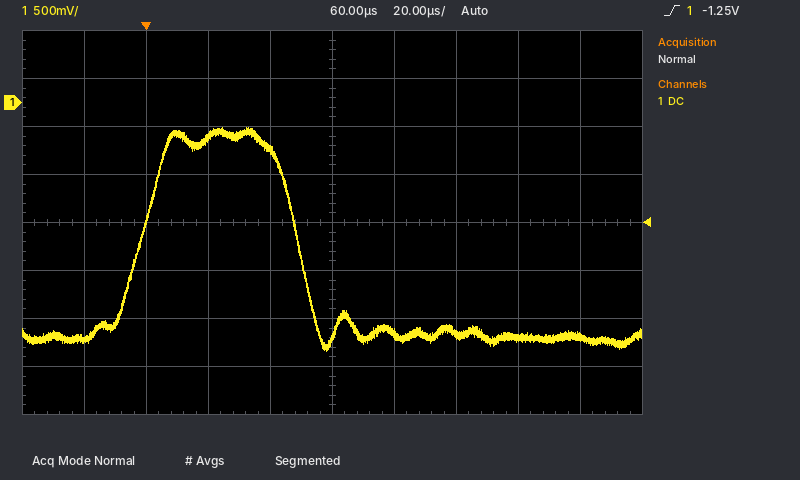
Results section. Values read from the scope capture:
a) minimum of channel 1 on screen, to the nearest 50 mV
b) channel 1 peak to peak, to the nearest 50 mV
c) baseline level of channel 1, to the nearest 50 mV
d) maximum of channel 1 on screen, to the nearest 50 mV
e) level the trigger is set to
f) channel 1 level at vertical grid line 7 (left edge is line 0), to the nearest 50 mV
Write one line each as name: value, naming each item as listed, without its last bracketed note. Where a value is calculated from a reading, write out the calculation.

minimum of channel 1 on screen, to the nearest 50 mV: -2.60 V
channel 1 peak to peak, to the nearest 50 mV: -250 mV − (-2.60 V) = 2.35 V
baseline level of channel 1, to the nearest 50 mV: -2.45 V
maximum of channel 1 on screen, to the nearest 50 mV: -250 mV
level the trigger is set to: -1.25 V
channel 1 level at vertical grid line 7 (left edge is line 0), to the nearest 50 mV: -2.40 V
